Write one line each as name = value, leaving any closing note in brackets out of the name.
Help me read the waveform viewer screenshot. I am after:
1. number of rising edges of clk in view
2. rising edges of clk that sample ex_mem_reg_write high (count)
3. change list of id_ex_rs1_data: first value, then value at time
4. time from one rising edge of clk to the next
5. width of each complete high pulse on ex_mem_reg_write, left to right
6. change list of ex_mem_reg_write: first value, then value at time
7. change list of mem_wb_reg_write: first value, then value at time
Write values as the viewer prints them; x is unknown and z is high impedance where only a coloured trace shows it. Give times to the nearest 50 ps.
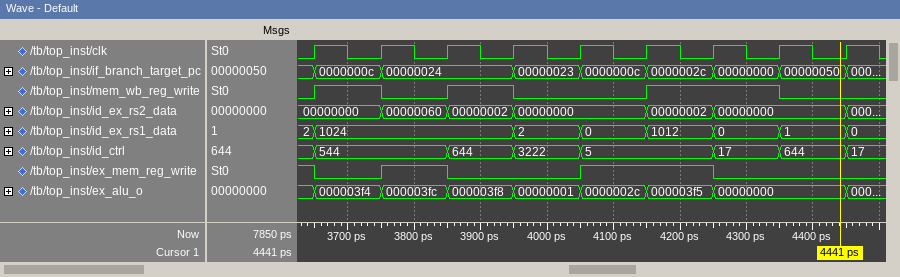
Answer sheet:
number of rising edges of clk in view = 9
rising edges of clk that sample ex_mem_reg_write high = 4
change list of id_ex_rs1_data: first value, then value at time = 2, 1024 at 3650 ps, 2 at 3950 ps, 0 at 4050 ps, 1012 at 4150 ps, 0 at 4250 ps, 1 at 4350 ps, 0 at 4450 ps
time from one rising edge of clk to the next = 100 ps
width of each complete high pulse on ex_mem_reg_write, left to right = 100 ps, 200 ps
change list of ex_mem_reg_write: first value, then value at time = 1, 0 at 3650 ps, 1 at 3750 ps, 0 at 3850 ps, 1 at 4050 ps, 0 at 4250 ps
change list of mem_wb_reg_write: first value, then value at time = 0, 1 at 3650 ps, 0 at 3750 ps, 1 at 3850 ps, 0 at 3950 ps, 1 at 4150 ps, 0 at 4350 ps
